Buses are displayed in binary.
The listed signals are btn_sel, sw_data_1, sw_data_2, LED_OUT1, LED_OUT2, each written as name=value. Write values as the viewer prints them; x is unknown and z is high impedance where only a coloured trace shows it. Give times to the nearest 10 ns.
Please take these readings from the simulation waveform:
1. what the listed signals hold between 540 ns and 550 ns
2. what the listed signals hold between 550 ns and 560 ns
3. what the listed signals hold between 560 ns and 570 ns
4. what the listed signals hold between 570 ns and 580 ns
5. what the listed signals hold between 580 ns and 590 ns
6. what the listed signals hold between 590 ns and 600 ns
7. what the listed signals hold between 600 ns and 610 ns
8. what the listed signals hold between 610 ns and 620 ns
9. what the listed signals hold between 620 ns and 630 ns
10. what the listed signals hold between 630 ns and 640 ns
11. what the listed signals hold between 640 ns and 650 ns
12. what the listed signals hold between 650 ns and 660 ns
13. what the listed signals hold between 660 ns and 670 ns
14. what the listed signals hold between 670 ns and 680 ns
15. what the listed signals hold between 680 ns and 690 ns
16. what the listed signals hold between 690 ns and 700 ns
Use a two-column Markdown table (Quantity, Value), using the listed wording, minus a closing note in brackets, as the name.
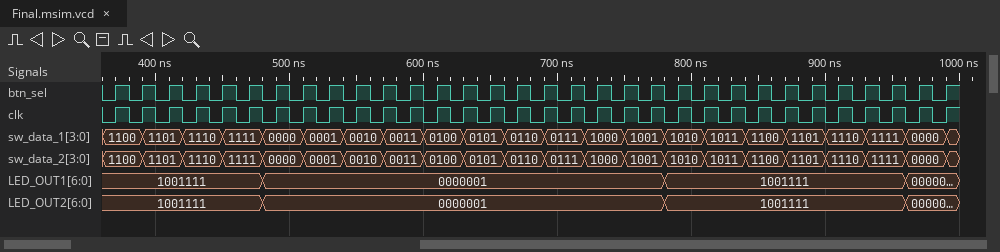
| Quantity | Value |
|---|---|
| what the listed signals hold between 540 ns and 550 ns | btn_sel=0, sw_data_1=0010, sw_data_2=0010, LED_OUT1=0000001, LED_OUT2=0000001 |
| what the listed signals hold between 550 ns and 560 ns | btn_sel=1, sw_data_1=0010, sw_data_2=0010, LED_OUT1=0000001, LED_OUT2=0000001 |
| what the listed signals hold between 560 ns and 570 ns | btn_sel=0, sw_data_1=0010, sw_data_2=0010, LED_OUT1=0000001, LED_OUT2=0000001 |
| what the listed signals hold between 570 ns and 580 ns | btn_sel=1, sw_data_1=0011, sw_data_2=0011, LED_OUT1=0000001, LED_OUT2=0000001 |
| what the listed signals hold between 580 ns and 590 ns | btn_sel=0, sw_data_1=0011, sw_data_2=0011, LED_OUT1=0000001, LED_OUT2=0000001 |
| what the listed signals hold between 590 ns and 600 ns | btn_sel=1, sw_data_1=0011, sw_data_2=0011, LED_OUT1=0000001, LED_OUT2=0000001 |
| what the listed signals hold between 600 ns and 610 ns | btn_sel=0, sw_data_1=0100, sw_data_2=0100, LED_OUT1=0000001, LED_OUT2=0000001 |
| what the listed signals hold between 610 ns and 620 ns | btn_sel=1, sw_data_1=0100, sw_data_2=0100, LED_OUT1=0000001, LED_OUT2=0000001 |
| what the listed signals hold between 620 ns and 630 ns | btn_sel=0, sw_data_1=0100, sw_data_2=0100, LED_OUT1=0000001, LED_OUT2=0000001 |
| what the listed signals hold between 630 ns and 640 ns | btn_sel=1, sw_data_1=0101, sw_data_2=0101, LED_OUT1=0000001, LED_OUT2=0000001 |
| what the listed signals hold between 640 ns and 650 ns | btn_sel=0, sw_data_1=0101, sw_data_2=0101, LED_OUT1=0000001, LED_OUT2=0000001 |
| what the listed signals hold between 650 ns and 660 ns | btn_sel=1, sw_data_1=0101, sw_data_2=0101, LED_OUT1=0000001, LED_OUT2=0000001 |
| what the listed signals hold between 660 ns and 670 ns | btn_sel=0, sw_data_1=0110, sw_data_2=0110, LED_OUT1=0000001, LED_OUT2=0000001 |
| what the listed signals hold between 670 ns and 680 ns | btn_sel=1, sw_data_1=0110, sw_data_2=0110, LED_OUT1=0000001, LED_OUT2=0000001 |
| what the listed signals hold between 680 ns and 690 ns | btn_sel=0, sw_data_1=0110, sw_data_2=0110, LED_OUT1=0000001, LED_OUT2=0000001 |
| what the listed signals hold between 690 ns and 700 ns | btn_sel=1, sw_data_1=0111, sw_data_2=0111, LED_OUT1=0000001, LED_OUT2=0000001 |
